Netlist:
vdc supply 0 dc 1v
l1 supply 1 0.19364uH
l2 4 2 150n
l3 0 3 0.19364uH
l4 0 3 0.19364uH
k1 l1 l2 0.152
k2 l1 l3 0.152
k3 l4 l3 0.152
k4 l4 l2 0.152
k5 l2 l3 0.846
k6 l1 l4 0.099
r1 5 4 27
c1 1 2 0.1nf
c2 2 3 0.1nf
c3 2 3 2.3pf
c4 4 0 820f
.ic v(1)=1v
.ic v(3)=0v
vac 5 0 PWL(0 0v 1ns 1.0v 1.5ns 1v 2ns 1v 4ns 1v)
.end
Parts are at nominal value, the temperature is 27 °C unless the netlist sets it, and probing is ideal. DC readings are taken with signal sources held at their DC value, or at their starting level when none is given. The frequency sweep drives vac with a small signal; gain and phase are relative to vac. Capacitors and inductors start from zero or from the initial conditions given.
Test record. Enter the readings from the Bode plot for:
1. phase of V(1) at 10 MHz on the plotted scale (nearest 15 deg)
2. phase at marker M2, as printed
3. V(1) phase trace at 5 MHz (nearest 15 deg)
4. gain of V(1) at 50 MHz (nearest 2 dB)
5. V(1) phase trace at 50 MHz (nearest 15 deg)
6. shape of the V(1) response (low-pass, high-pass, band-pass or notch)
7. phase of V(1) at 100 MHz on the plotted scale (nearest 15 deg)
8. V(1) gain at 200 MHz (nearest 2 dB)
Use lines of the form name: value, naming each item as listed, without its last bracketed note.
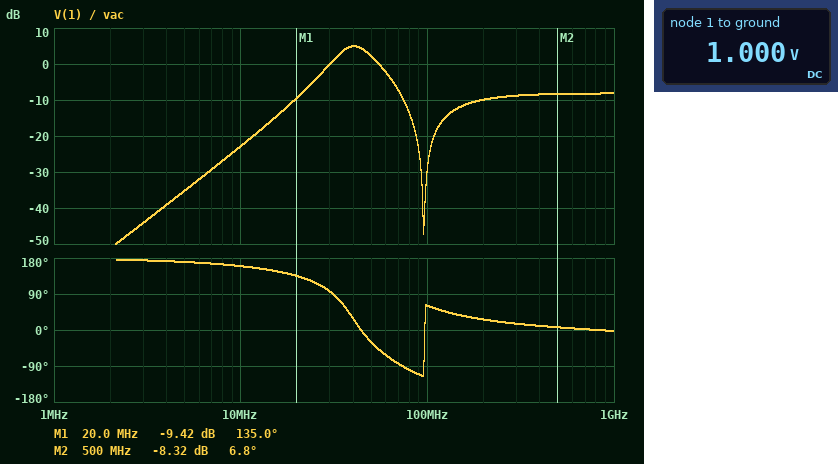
phase of V(1) at 10 MHz on the plotted scale: 165 deg
phase at marker M2, as printed: 6.8 deg
V(1) phase trace at 5 MHz: 165 deg
gain of V(1) at 50 MHz: 2 dB
V(1) phase trace at 50 MHz: -30 deg
shape of the V(1) response: band-pass
phase of V(1) at 100 MHz on the plotted scale: 60 deg
V(1) gain at 200 MHz: -10 dB
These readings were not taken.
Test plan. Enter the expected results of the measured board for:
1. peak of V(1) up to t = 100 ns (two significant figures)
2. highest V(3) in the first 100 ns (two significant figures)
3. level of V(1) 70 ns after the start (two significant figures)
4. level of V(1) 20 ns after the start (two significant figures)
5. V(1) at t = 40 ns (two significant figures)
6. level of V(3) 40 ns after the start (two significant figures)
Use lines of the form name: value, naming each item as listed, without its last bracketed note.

peak of V(1) up to t = 100 ns: 1.3 V
highest V(3) in the first 100 ns: 280 mV
level of V(1) 70 ns after the start: 980 mV
level of V(1) 20 ns after the start: 710 mV
V(1) at t = 40 ns: 920 mV
level of V(3) 40 ns after the start: 43 mV
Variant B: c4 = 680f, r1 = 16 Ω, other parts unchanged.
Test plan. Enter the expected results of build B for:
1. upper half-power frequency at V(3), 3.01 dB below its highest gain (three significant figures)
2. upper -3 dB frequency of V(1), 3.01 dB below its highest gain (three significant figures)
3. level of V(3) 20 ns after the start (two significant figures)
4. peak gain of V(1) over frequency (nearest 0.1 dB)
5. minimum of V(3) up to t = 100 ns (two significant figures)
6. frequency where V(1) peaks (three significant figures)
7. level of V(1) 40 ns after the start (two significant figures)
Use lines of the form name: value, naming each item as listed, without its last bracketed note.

upper half-power frequency at V(3), 3.01 dB below its highest gain: 96.9 MHz
upper -3 dB frequency of V(1), 3.01 dB below its highest gain: 46.2 MHz
level of V(3) 20 ns after the start: 68 mV
peak gain of V(1) over frequency: 6.9 dB
minimum of V(3) up to t = 100 ns: -360 mV
frequency where V(1) peaks: 34.9 MHz
level of V(1) 40 ns after the start: 970 mV
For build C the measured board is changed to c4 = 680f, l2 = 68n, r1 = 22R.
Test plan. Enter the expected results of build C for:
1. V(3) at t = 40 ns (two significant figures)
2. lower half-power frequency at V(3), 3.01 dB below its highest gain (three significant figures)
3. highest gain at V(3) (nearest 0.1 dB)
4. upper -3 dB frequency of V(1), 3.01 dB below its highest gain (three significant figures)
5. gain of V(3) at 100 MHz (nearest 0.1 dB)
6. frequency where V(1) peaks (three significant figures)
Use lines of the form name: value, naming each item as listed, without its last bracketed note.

V(3) at t = 40 ns: 72 mV
lower half-power frequency at V(3), 3.01 dB below its highest gain: 39.7 MHz
highest gain at V(3): 1.3 dB
upper -3 dB frequency of V(1), 3.01 dB below its highest gain: 46.1 MHz
gain of V(3) at 100 MHz: 1.2 dB
frequency where V(1) peaks: 40.2 MHz
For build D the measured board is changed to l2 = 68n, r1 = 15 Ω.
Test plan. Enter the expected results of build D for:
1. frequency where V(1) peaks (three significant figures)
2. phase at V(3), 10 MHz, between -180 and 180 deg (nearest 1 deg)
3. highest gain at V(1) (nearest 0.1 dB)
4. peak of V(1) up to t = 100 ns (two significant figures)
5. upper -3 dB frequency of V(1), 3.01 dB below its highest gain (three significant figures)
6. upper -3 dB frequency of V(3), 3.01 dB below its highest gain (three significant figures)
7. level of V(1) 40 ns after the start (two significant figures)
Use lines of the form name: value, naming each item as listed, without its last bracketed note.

frequency where V(1) peaks: 37.7 MHz
phase at V(3), 10 MHz, between -180 and 180 deg: 169 deg
highest gain at V(1): 9.7 dB
peak of V(1) up to t = 100 ns: 1.8 V
upper -3 dB frequency of V(1), 3.01 dB below its highest gain: 43.7 MHz
upper -3 dB frequency of V(3), 3.01 dB below its highest gain: 169 MHz
level of V(1) 40 ns after the start: 800 mV
